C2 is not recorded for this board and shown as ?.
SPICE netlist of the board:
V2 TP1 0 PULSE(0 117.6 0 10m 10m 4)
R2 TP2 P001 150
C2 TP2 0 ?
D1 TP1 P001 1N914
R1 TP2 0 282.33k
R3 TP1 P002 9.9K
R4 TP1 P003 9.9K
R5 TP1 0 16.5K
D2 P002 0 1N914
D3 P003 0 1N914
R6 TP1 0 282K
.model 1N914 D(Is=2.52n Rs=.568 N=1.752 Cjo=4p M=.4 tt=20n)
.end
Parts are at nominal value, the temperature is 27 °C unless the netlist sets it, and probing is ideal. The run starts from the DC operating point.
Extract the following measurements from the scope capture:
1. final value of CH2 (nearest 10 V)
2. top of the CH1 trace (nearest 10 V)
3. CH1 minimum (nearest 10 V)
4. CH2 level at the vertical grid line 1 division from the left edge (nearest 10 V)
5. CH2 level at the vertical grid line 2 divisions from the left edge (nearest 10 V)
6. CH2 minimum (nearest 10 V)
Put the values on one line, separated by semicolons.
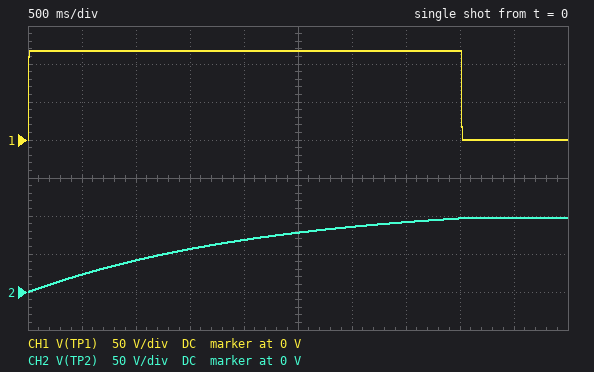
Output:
100 V; 120 V; 0 V; 20 V; 40 V; 0 V
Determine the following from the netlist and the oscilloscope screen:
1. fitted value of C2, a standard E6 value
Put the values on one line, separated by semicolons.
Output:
15 mF
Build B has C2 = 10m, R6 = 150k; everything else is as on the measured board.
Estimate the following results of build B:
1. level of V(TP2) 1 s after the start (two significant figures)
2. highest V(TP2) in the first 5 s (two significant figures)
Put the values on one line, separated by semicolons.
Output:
56 V; 110 V
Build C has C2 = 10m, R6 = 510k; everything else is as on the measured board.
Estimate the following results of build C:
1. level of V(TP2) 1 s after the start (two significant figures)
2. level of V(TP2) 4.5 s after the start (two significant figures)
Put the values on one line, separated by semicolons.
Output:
56 V; 110 V
